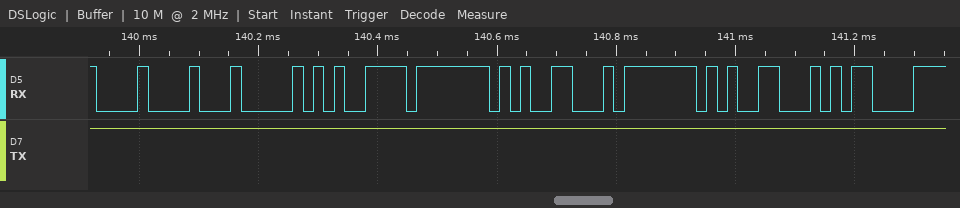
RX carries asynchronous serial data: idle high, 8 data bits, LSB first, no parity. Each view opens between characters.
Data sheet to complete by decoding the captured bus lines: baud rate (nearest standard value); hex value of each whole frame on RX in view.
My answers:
57600 baud
08, 04, E5, 7F, 19, 7F, 19, 0D
